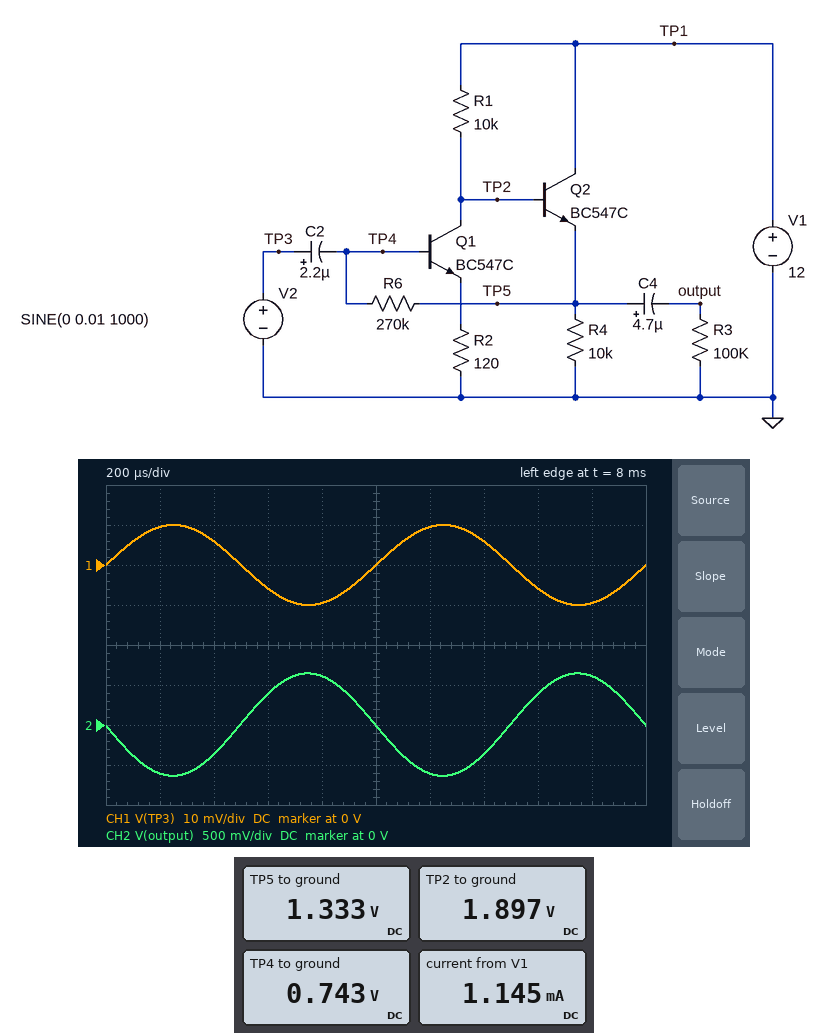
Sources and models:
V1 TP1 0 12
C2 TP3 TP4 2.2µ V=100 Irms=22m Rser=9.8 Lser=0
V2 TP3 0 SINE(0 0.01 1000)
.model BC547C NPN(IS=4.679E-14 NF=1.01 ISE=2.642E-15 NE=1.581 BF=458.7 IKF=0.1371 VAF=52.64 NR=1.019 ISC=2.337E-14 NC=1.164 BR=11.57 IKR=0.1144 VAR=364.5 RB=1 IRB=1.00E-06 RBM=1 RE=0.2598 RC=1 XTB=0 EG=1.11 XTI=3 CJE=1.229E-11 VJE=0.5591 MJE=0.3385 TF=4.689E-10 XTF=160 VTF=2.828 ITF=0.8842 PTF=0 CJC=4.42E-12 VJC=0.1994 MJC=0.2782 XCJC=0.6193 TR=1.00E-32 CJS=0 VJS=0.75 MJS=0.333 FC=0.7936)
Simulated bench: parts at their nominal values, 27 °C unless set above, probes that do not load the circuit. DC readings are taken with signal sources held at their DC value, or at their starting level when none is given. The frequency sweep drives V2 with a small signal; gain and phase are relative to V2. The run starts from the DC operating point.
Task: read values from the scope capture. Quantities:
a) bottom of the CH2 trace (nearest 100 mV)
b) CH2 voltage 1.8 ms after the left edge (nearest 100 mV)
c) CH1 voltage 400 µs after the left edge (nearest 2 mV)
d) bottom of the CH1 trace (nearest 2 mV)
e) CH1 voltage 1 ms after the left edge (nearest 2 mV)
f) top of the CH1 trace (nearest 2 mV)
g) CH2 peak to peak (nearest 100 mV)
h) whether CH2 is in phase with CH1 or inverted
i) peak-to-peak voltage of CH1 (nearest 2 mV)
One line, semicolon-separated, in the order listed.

-600 mV; 600 mV; 6 mV; -10 mV; 0 V; 10 mV; 1.3 V; inverted; 20 mV
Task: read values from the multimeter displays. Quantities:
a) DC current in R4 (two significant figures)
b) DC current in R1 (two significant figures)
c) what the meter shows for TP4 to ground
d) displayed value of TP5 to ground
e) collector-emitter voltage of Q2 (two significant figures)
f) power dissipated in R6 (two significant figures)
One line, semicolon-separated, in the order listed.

130 µA; 1.0 mA; 0.743 V; 1.333 V; 11 V; 1.3 µW
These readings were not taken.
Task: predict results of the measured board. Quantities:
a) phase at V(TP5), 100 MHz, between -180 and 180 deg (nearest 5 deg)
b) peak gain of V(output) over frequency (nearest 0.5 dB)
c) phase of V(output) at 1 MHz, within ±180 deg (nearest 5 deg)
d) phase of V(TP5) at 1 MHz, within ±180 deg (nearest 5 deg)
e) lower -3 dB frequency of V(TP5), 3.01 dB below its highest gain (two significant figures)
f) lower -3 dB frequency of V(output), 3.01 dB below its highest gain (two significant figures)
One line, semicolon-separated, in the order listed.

50 deg; 36.0 dB; 165 deg; 165 deg; 19 Hz; 19 Hz
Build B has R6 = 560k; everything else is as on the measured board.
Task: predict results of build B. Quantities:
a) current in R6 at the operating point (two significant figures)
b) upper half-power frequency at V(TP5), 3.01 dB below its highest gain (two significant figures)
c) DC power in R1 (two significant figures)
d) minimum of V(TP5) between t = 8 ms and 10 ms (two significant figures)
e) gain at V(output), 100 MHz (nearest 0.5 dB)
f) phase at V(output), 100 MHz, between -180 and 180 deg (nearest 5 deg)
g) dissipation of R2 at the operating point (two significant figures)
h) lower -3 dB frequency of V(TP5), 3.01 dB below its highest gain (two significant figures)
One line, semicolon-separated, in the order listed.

2.0 µA; 3.6 MHz; 9.1 mW; 1.2 V; 8.0 dB; 50 deg; 110 µW; 9.6 Hz
